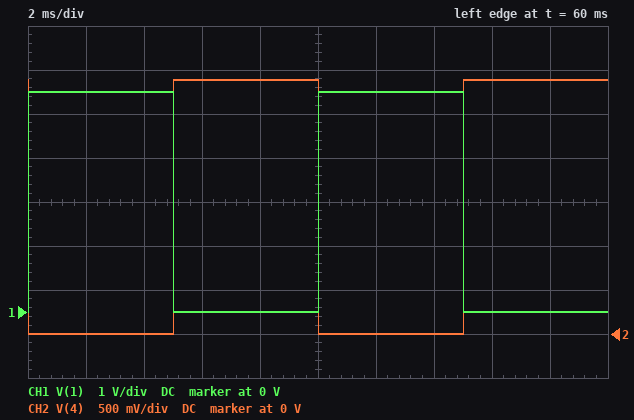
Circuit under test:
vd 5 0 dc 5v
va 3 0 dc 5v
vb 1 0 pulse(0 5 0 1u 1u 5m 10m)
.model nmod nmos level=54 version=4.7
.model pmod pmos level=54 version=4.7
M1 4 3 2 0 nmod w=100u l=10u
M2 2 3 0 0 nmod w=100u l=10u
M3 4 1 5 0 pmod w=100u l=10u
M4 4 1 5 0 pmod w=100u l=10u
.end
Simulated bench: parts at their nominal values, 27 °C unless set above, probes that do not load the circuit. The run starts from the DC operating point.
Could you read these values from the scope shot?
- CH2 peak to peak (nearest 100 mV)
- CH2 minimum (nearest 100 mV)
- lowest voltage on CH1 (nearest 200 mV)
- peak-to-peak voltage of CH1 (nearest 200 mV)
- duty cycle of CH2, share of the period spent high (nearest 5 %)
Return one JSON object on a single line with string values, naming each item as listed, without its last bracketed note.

{"CH2 peak to peak": "2.9 V", "CH2 minimum": "0 V", "lowest voltage on CH1": "0 V", "peak-to-peak voltage of CH1": "5.0 V", "duty cycle of CH2, share of the period spent high": "50 %"}
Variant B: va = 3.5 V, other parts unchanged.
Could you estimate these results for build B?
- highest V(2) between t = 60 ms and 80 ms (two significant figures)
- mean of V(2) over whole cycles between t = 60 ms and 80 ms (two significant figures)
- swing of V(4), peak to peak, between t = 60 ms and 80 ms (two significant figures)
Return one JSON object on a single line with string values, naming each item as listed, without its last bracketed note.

{"highest V(2) between t = 60 ms and 80 ms": "1.0 V", "mean of V(2) over whole cycles between t = 60 ms and 80 ms": "510 mV", "swing of V(4), peak to peak, between t = 60 ms and 80 ms": "3.9 V"}
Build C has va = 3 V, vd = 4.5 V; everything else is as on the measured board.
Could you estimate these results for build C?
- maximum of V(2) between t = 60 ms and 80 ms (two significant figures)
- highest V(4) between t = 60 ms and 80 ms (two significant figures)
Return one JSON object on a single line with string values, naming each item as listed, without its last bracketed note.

{"maximum of V(2) between t = 60 ms and 80 ms": "850 mV", "highest V(4) between t = 60 ms and 80 ms": "3.6 V"}
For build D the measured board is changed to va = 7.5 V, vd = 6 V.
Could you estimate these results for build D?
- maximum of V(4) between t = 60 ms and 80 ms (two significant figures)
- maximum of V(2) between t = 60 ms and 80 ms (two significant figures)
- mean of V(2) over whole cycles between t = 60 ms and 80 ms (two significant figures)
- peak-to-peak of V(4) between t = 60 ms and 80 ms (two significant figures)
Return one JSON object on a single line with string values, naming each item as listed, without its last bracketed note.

{"maximum of V(4) between t = 60 ms and 80 ms": "3.0 V", "maximum of V(2) between t = 60 ms and 80 ms": "1.4 V", "mean of V(2) over whole cycles between t = 60 ms and 80 ms": "750 mV", "peak-to-peak of V(4) between t = 60 ms and 80 ms": "2.7 V"}
